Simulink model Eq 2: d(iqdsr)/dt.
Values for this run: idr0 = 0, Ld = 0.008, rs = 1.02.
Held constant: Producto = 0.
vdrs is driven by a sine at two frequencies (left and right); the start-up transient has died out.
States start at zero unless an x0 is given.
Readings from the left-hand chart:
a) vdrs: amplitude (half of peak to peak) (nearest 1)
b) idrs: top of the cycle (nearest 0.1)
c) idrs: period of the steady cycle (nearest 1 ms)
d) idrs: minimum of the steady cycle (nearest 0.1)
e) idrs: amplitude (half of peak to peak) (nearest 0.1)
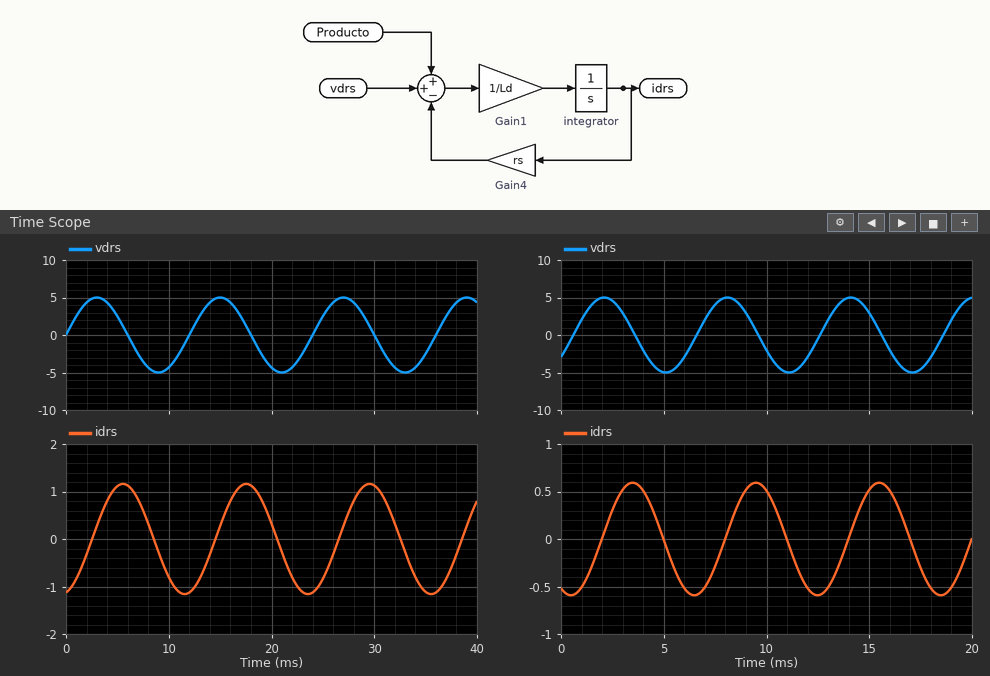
5
1.2
12 ms
-1.2
1.2
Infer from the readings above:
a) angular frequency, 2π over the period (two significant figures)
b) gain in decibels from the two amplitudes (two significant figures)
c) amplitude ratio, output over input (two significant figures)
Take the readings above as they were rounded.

0.52 rad/ms
-12 dB
0.24
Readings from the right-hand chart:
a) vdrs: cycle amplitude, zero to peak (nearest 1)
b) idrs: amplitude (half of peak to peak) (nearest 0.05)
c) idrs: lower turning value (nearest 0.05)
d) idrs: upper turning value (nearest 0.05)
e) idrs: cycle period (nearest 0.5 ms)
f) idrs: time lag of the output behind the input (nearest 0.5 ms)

5
0.60
-0.60
0.60
6.0 ms
1.5 ms
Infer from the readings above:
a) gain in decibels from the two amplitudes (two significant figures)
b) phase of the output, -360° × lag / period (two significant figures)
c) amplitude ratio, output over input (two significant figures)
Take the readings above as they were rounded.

-18 dB
-90°
0.12
